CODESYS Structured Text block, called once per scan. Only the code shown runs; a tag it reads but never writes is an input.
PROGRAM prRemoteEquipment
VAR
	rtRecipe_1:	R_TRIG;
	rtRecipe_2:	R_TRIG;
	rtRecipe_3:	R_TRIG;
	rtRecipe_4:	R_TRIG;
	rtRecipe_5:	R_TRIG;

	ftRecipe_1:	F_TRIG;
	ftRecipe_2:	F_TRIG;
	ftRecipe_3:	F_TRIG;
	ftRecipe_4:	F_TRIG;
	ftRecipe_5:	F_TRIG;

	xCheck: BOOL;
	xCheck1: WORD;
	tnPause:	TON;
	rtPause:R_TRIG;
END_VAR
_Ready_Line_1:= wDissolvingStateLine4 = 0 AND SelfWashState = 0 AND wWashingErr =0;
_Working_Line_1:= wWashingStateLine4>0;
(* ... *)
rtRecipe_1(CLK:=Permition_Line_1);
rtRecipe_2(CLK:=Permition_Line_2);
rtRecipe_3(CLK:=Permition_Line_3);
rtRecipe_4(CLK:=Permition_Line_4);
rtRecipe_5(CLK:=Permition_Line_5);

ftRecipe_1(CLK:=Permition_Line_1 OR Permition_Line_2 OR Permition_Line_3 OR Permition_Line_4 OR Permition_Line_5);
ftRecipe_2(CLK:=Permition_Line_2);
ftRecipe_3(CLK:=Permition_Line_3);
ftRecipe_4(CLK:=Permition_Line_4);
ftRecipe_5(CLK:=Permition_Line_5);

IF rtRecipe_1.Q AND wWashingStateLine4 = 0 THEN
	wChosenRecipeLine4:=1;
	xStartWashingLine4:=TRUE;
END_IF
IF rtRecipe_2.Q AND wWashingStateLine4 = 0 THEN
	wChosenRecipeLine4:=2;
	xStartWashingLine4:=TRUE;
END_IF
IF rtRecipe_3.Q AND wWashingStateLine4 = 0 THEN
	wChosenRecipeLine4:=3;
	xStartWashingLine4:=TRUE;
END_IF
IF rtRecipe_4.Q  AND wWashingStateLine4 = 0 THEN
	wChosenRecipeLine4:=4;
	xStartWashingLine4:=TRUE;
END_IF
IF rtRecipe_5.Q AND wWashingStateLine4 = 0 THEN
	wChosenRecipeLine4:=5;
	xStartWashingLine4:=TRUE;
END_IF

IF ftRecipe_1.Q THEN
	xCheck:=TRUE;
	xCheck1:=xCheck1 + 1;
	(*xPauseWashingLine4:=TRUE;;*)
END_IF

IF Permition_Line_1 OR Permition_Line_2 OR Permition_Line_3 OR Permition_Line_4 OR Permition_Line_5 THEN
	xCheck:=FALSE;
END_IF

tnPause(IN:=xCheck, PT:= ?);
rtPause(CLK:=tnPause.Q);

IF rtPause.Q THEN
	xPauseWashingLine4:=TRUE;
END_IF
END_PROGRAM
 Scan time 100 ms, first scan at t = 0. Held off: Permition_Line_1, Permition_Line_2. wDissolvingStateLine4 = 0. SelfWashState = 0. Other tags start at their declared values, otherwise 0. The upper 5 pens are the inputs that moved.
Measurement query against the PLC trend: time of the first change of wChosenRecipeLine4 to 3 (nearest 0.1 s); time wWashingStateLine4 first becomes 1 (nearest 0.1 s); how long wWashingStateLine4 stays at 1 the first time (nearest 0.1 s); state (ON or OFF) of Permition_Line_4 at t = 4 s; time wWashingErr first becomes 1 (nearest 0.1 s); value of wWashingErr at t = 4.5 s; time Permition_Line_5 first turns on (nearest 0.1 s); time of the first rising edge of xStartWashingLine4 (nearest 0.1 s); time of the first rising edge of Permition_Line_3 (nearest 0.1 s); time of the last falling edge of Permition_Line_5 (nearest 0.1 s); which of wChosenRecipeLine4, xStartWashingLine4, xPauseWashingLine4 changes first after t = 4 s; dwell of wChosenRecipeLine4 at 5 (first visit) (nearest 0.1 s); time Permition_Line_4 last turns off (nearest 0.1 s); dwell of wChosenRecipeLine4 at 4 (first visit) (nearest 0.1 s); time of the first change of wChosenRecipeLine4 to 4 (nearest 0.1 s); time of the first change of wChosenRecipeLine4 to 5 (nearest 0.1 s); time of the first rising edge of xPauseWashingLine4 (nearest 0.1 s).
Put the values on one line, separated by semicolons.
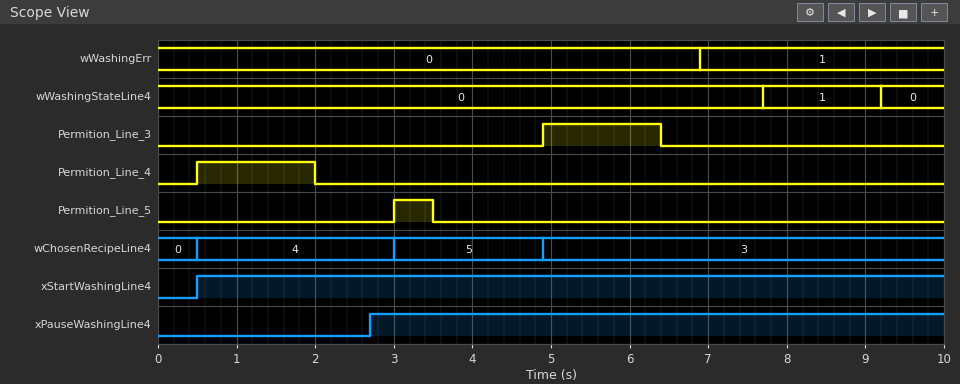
4.9 s; 7.7 s; 1.5 s; OFF; 6.9 s; 0; 3.0 s; 0.5 s; 4.9 s; 3.5 s; wChosenRecipeLine4; 1.9 s; 2.0 s; 2.5 s; 0.5 s; 3.0 s; 2.7 s
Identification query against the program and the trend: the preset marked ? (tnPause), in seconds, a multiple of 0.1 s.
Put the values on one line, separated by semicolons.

0.7 s
